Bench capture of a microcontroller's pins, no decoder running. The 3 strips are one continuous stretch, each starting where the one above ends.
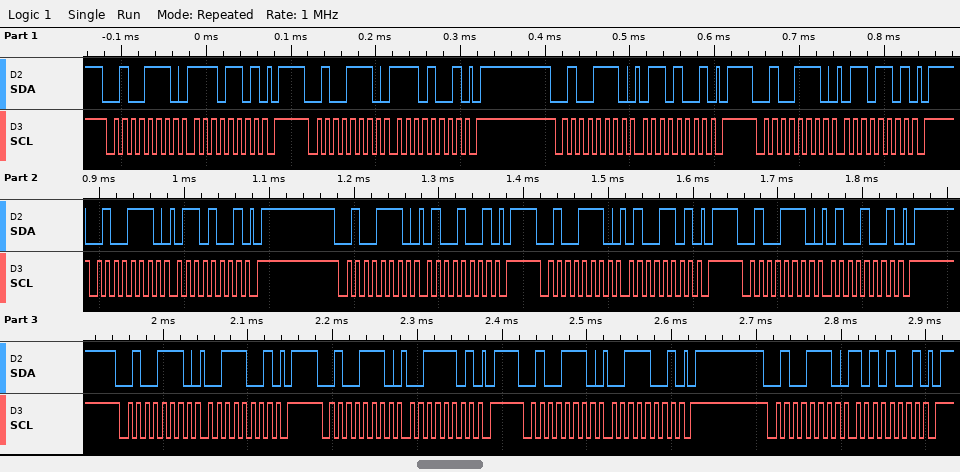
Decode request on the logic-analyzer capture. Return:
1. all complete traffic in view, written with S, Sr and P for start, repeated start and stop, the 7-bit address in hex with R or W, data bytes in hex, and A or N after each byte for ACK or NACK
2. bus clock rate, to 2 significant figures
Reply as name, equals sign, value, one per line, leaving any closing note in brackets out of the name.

all complete traffic in view, written with S, Sr and P for start, repeated start and stop, the 7-bit address in hex with R or W, data bytes in hex, and A or N after each byte for ACK or NACK = S 27W A ED A P S 27W A E9 A P S 27W A 69 A P S 27W A 6D A P S 27W A 69 A P S 27W A 49 A P S 27W A 4D A P S 27W A 49 A P S 27W A 39 A P S 27W A 3D A P S 27W A 39 A P S 27W A A9 A P
bus clock rate, to 2 significant figures = 100 kHz
